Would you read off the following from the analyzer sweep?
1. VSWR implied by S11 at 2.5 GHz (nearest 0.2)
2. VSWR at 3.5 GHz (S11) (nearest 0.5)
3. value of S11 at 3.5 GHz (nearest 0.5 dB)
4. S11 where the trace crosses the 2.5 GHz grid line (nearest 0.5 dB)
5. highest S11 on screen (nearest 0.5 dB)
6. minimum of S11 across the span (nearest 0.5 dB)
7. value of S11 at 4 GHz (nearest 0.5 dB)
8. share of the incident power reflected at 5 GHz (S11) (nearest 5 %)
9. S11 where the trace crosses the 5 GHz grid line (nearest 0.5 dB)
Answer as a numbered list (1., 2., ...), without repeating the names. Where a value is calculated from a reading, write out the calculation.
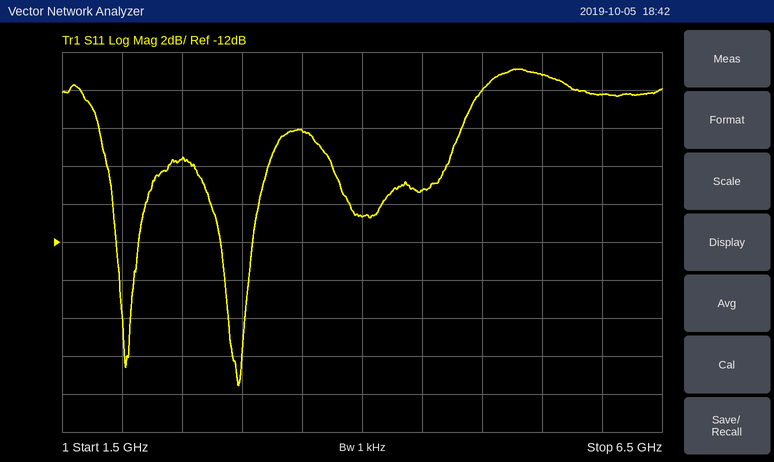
1. |Γ| = 10^(-7.5/20) = 0.4217; VSWR = (1 + 0.4217)/(1 − 0.4217) ≈ 2.46, so 2.4 to the nearest 0.2
2. |Γ| = 10^(-6/20) = 0.5012; VSWR = (1 + 0.5012)/(1 − 0.5012) ≈ 3.0
3. -6.0 dB
4. -7.5 dB
5. -3.0 dB
6. -19.5 dB
7. -10.5 dB
8. 10^(-4/10) ≈ 40 %
9. -4.0 dB
